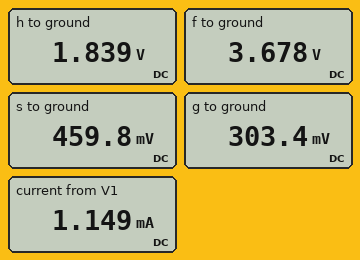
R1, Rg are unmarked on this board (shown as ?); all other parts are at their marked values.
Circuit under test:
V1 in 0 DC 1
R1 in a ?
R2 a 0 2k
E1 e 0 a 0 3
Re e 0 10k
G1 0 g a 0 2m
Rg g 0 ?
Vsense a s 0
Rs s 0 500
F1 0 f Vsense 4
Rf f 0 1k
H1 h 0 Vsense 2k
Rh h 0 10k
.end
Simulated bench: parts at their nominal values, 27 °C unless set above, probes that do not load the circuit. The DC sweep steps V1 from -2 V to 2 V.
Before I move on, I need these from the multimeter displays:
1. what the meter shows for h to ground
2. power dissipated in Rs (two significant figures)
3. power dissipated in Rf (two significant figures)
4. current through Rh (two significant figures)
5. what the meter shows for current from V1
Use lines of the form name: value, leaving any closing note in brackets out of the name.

what the meter shows for h to ground: 1.839 V
power dissipated in Rs: 420 µW
power dissipated in Rf: 14 mW
current through Rh: 180 µA
what the meter shows for current from V1: 1.149 mA
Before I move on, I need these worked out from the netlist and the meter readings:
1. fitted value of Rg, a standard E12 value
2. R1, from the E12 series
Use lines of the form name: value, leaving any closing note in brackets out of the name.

fitted value of Rg, a standard E12 value: 330 Ω
R1, from the E12 series: 470 Ω
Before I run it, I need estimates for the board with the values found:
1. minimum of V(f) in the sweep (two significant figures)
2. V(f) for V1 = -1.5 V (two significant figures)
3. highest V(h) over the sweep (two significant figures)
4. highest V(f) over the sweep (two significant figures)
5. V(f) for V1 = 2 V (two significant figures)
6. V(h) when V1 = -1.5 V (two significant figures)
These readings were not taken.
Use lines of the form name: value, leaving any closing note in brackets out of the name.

minimum of V(f) in the sweep: -7.4 V
V(f) for V1 = -1.5 V: -5.5 V
highest V(h) over the sweep: 3.7 V
highest V(f) over the sweep: 7.4 V
V(f) for V1 = 2 V: 7.4 V
V(h) when V1 = -1.5 V: -2.8 V
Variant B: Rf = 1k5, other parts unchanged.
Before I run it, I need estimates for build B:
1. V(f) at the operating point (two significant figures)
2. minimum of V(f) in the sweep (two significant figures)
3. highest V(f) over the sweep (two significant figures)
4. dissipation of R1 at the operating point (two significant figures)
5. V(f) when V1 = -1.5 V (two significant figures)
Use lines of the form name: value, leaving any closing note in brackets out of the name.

V(f) at the operating point: 5.5 V
minimum of V(f) in the sweep: -11 V
highest V(f) over the sweep: 11 V
dissipation of R1 at the operating point: 620 µW
V(f) when V1 = -1.5 V: -8.3 V
